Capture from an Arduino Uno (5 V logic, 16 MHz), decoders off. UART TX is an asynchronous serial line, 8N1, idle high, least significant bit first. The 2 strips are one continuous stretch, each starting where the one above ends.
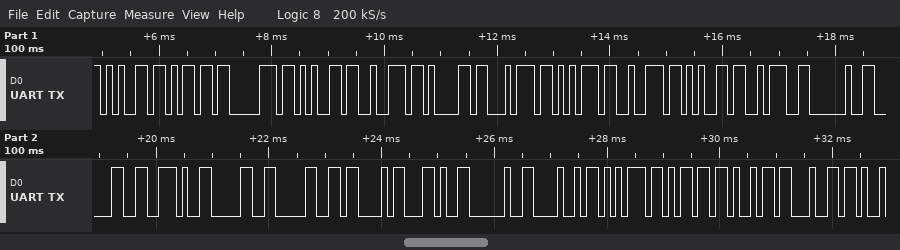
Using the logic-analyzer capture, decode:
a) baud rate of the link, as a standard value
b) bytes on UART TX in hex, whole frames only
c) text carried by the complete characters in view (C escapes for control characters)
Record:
9600 baud
65 6D 70 65 72 61 74 75 72 65 3A 20 30 2E 30 30 43 2C 20 48 75 6D 69 64
"emperature: 0.00C, Humid"
